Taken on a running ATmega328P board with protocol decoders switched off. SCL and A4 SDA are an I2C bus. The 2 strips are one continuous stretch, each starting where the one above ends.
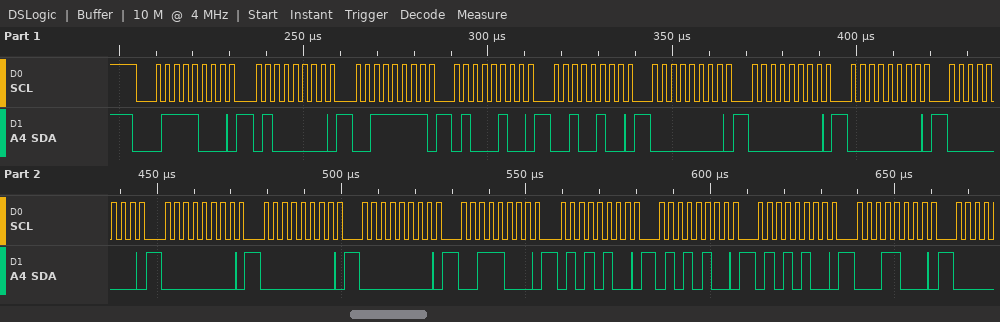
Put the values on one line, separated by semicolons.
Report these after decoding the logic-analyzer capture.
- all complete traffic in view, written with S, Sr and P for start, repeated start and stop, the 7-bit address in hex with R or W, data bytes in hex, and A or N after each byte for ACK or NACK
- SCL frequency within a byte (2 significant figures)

S 3CW A 40 A 3F A 44 A 24 A 00 A 00 A 00 A 00 A 00 A 00 A 00 A 38 A 54 A 54 A 54 A 18 A; 400 kHz
